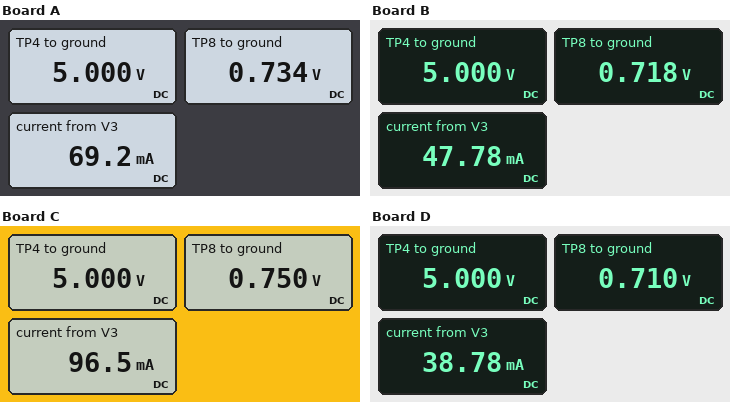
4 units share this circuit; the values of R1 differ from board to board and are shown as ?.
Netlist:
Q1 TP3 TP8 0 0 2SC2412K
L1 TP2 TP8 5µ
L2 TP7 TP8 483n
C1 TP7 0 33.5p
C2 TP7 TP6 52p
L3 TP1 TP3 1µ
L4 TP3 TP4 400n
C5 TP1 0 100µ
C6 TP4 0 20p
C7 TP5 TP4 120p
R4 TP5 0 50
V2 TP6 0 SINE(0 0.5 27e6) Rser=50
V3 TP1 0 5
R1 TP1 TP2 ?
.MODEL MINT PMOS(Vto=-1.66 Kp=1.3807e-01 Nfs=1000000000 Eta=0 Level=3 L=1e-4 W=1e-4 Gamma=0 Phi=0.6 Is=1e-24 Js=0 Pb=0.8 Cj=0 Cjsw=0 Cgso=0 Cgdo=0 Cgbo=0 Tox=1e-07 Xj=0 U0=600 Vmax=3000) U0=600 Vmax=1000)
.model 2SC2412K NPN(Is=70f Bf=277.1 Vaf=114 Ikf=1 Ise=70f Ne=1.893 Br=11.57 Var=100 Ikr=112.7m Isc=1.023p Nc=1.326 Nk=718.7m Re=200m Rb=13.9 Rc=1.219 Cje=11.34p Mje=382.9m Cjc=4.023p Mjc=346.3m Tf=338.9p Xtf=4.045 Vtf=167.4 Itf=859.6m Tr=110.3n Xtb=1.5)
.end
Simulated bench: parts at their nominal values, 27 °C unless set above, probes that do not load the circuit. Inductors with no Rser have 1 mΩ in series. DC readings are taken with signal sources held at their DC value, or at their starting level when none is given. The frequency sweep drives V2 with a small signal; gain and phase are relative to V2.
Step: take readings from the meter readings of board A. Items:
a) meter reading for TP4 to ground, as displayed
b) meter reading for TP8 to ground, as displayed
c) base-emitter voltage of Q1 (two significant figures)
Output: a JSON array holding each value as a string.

["5.000 V", "0.734 V", "730 mV"]
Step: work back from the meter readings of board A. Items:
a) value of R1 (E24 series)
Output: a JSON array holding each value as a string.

["16 kΩ"]
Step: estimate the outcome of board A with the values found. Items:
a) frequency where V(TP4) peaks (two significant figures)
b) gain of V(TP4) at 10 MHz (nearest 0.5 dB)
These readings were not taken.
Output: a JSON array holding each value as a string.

["11 MHz", "24.5 dB"]
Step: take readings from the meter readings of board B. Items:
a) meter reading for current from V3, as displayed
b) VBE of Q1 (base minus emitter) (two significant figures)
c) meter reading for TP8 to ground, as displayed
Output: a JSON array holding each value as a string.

["47.78 mA", "720 mV", "0.718 V"]
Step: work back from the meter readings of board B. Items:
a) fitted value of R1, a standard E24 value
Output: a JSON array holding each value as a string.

["24 kΩ"]
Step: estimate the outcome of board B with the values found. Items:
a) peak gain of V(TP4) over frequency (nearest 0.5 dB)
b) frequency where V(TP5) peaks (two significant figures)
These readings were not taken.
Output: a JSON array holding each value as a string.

["25.0 dB", "26 MHz"]
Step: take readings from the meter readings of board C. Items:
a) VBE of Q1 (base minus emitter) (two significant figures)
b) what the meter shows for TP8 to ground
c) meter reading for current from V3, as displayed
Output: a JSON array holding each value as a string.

["750 mV", "0.750 V", "96.5 mA"]
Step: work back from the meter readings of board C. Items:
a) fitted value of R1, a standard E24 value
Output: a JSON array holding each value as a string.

["11 kΩ"]
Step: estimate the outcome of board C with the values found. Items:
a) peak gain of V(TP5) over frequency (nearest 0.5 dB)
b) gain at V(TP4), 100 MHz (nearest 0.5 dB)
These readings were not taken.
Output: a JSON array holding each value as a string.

["19.5 dB", "-15.5 dB"]
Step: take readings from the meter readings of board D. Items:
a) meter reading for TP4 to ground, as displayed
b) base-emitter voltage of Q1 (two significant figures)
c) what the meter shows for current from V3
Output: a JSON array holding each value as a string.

["5.000 V", "710 mV", "38.78 mA"]
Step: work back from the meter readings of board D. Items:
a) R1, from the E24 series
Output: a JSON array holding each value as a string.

["30 kΩ"]
